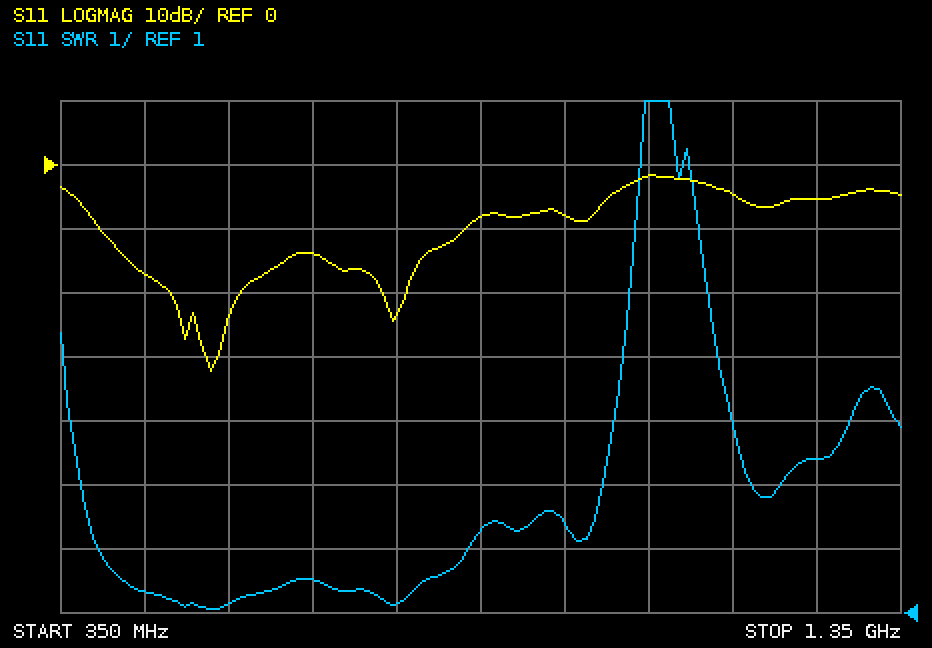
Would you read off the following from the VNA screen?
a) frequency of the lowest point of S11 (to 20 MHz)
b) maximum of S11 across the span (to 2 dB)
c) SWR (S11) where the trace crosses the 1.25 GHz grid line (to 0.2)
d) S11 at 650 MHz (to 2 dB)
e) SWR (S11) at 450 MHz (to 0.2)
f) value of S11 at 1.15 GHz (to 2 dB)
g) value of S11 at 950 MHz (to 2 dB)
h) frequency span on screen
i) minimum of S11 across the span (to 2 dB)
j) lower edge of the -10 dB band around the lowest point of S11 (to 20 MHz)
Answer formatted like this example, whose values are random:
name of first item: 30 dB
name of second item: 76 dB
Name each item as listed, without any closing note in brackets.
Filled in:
frequency of the lowest point of S11: 520 MHz
maximum of S11 across the span: -2 dB
SWR (S11) where the trace crosses the 1.25 GHz grid line: 3.4
S11 at 650 MHz: -14 dB
SWR (S11) at 450 MHz: 1.4
value of S11 at 1.15 GHz: -4 dB
value of S11 at 950 MHz: -8 dB
frequency span on screen: 1 GHz
minimum of S11 across the span: -32 dB
lower edge of the -10 dB band around the lowest point of S11: 400 MHz
